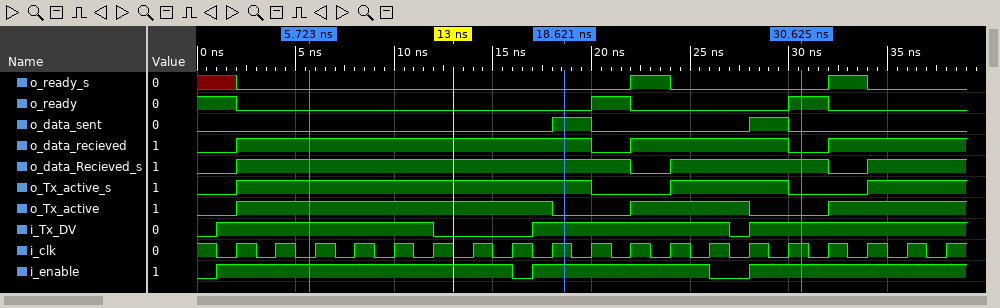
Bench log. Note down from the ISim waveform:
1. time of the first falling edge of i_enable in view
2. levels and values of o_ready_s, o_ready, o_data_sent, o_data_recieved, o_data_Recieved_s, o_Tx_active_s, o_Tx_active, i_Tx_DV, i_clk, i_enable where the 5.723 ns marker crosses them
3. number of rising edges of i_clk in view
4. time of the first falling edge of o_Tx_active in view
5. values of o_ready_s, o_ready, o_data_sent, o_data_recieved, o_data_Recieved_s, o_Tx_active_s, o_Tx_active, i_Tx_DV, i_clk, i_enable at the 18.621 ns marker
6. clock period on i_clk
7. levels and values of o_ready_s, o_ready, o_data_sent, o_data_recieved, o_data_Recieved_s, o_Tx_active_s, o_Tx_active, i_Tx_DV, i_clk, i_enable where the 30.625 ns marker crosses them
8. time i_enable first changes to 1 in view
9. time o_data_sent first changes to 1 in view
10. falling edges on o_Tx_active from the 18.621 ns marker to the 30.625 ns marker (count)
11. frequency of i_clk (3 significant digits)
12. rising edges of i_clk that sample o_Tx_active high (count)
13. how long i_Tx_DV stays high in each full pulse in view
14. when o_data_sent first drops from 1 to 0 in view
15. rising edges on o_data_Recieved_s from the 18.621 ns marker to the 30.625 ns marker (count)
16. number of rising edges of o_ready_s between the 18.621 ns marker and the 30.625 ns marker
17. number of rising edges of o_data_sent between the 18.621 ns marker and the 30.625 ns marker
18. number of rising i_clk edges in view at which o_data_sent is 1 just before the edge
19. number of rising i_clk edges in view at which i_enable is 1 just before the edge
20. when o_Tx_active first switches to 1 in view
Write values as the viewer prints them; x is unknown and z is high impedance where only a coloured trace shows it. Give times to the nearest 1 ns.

16 ns
o_ready_s=0, o_ready=0, o_data_sent=0, o_data_recieved=1, o_data_Recieved_s=1, o_Tx_active_s=1, o_Tx_active=1, i_Tx_DV=1, i_clk=0, i_enable=1
19
18 ns
o_ready_s=0, o_ready=0, o_data_sent=1, o_data_recieved=1, o_data_Recieved_s=1, o_Tx_active_s=1, o_Tx_active=0, i_Tx_DV=1, i_clk=1, i_enable=1
2 ns
o_ready_s=0, o_ready=1, o_data_sent=0, o_data_recieved=0, o_data_Recieved_s=1, o_Tx_active_s=0, o_Tx_active=0, i_Tx_DV=1, i_clk=1, i_enable=1
1 ns
18 ns
1
500 MHz
14
11 ns, 10 ns
20 ns
1
1
1
2
18
2 ns
